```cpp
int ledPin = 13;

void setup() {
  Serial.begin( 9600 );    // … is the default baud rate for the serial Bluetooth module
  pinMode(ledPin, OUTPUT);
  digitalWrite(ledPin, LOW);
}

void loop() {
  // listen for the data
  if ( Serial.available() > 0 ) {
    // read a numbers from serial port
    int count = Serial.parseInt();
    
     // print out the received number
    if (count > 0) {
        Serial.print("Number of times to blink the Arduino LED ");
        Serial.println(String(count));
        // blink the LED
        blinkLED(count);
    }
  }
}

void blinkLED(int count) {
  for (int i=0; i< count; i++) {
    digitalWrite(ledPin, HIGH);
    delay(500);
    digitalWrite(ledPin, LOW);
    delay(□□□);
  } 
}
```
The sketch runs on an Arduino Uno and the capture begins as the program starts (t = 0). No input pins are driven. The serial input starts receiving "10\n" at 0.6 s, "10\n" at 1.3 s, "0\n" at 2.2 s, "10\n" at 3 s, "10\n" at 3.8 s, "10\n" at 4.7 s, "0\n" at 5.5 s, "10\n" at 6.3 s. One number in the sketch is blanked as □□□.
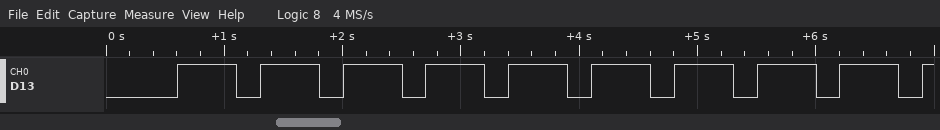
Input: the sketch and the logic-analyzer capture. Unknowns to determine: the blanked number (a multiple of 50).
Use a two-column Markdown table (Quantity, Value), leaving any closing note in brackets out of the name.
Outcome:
| Quantity | Value |
|---|---|
| the blanked number | 200 |
